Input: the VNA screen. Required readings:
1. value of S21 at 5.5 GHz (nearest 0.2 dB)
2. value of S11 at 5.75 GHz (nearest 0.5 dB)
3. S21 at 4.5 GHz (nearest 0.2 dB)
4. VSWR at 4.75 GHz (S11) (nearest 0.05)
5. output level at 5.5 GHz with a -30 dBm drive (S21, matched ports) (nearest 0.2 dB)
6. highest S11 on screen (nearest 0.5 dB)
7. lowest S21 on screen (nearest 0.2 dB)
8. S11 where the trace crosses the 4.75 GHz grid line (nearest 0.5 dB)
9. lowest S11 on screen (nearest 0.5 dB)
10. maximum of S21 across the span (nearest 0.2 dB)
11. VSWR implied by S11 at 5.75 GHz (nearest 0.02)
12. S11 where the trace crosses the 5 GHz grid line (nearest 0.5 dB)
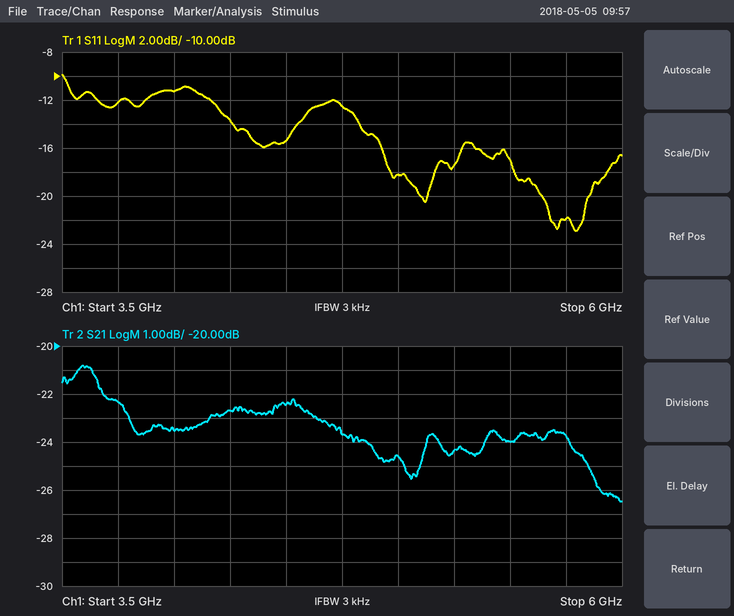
-24.0 dB
-22.0 dB
-22.4 dB
1.60
-54.0 dBm
-10.0 dB
-26.4 dB
-12.5 dB
-23.0 dB
-20.8 dB
1.18
-18.0 dB
